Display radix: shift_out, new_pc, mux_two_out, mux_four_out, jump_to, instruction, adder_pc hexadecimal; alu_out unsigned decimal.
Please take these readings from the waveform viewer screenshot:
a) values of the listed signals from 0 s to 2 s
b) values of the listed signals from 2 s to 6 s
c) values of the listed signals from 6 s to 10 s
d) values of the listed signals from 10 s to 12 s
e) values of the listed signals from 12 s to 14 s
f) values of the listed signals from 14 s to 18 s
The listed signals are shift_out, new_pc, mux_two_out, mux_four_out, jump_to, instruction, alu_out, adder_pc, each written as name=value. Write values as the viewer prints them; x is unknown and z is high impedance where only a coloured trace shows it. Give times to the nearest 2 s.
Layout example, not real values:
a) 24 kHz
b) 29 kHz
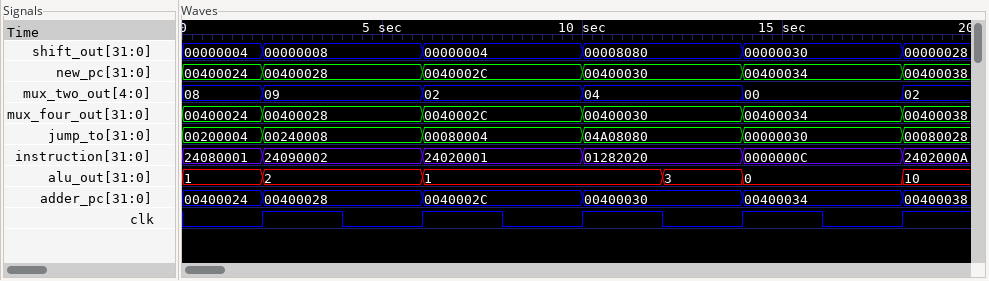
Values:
a) shift_out=00000004, new_pc=00400024, mux_two_out=08, mux_four_out=00400024, jump_to=00200004, instruction=24080001, alu_out=1, adder_pc=00400024
b) shift_out=00000008, new_pc=00400028, mux_two_out=09, mux_four_out=00400028, jump_to=00240008, instruction=24090002, alu_out=2, adder_pc=00400028
c) shift_out=00000004, new_pc=0040002C, mux_two_out=02, mux_four_out=0040002C, jump_to=00080004, instruction=24020001, alu_out=1, adder_pc=0040002C
d) shift_out=00008080, new_pc=00400030, mux_two_out=04, mux_four_out=00400030, jump_to=04A08080, instruction=01282020, alu_out=1, adder_pc=00400030
e) shift_out=00008080, new_pc=00400030, mux_two_out=04, mux_four_out=00400030, jump_to=04A08080, instruction=01282020, alu_out=3, adder_pc=00400030
f) shift_out=00000030, new_pc=00400034, mux_two_out=00, mux_four_out=00400034, jump_to=00000030, instruction=0000000C, alu_out=0, adder_pc=00400034
